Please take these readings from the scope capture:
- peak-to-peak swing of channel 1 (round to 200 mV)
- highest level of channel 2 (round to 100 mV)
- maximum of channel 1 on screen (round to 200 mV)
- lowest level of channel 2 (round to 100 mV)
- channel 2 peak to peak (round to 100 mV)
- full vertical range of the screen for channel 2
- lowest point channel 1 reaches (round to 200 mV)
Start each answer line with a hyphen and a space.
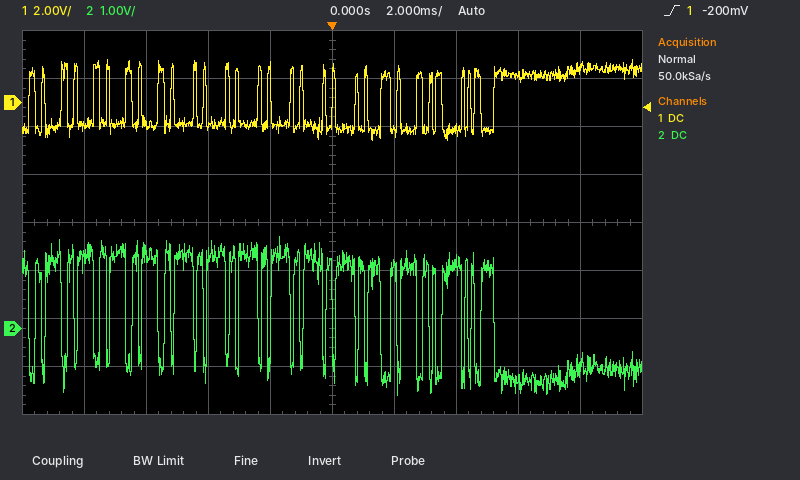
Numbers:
- 3.4 V
- 1.9 V
- 1.8 V
- -1.4 V
- 3.3 V
- 8 V
- -1.6 V
